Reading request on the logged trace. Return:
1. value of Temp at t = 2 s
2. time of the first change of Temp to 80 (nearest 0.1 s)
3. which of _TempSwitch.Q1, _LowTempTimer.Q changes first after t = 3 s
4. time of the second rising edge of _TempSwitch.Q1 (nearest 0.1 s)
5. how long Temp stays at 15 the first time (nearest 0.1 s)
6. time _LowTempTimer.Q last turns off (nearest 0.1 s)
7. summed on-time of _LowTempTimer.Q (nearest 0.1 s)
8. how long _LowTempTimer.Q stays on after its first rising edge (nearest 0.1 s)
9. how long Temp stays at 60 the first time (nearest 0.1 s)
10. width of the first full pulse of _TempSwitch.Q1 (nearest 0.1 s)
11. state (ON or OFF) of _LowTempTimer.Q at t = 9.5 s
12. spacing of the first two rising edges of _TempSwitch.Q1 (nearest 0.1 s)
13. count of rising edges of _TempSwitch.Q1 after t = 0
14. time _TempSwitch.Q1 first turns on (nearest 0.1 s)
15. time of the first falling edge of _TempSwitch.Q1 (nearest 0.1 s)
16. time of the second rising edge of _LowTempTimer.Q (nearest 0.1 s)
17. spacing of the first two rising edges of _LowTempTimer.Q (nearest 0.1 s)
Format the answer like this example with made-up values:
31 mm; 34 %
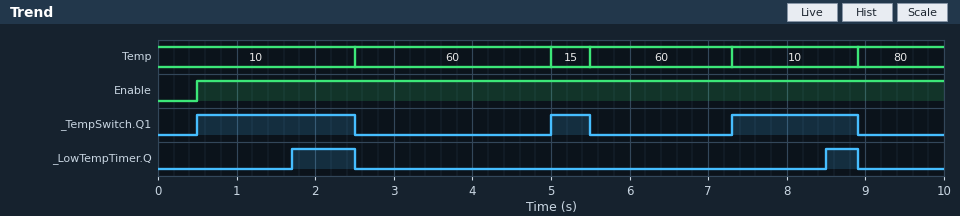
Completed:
10; 8.9 s; _TempSwitch.Q1; 5.0 s; 0.5 s; 8.9 s; 1.2 s; 0.8 s; 2.5 s; 2.0 s; OFF; 4.5 s; 3; 0.5 s; 2.5 s; 8.5 s; 6.8 s
